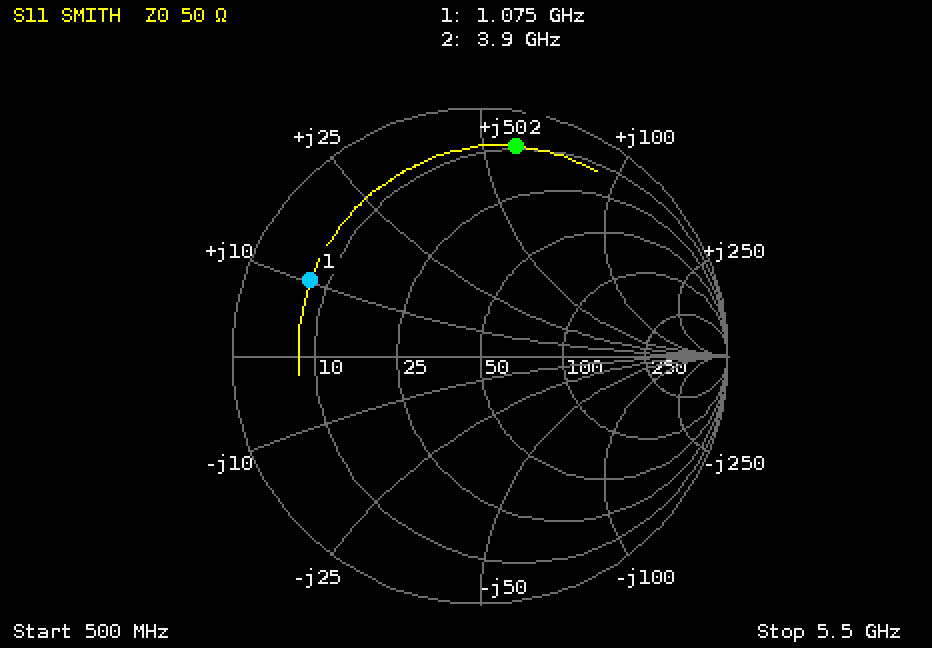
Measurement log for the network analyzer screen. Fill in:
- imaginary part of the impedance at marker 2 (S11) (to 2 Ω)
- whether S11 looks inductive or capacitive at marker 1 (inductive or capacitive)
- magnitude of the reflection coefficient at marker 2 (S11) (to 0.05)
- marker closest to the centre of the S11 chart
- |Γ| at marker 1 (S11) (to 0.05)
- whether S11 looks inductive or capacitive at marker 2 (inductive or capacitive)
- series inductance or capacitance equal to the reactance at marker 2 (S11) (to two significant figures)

+58 Ω
inductive
0.85
marker 1
0.75
inductive
2.4 nH
